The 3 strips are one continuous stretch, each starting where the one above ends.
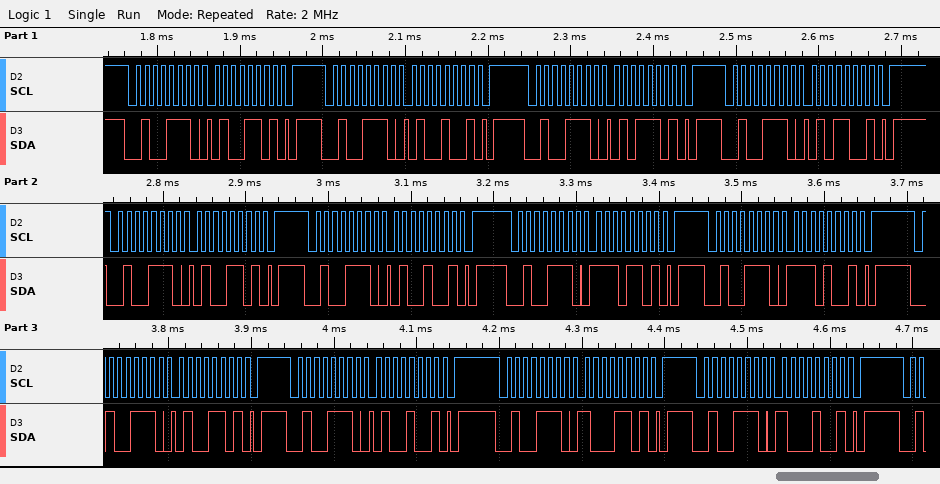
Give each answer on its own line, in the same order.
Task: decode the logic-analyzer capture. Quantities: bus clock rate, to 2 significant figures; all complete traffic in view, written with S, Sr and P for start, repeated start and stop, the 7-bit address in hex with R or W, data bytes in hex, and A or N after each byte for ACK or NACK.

100 kHz
S 27W A 4D A P S 27W A 49 A P S 27W A 5D A P S 27W A 59 A P S 27W A 4D A P S 27W A 49 A P S 27W A ED A P S 27W A E9 A P S 27W A 4D A P S 27W A 49 A P S 27W A 8D A P S 27W A 89 A P
